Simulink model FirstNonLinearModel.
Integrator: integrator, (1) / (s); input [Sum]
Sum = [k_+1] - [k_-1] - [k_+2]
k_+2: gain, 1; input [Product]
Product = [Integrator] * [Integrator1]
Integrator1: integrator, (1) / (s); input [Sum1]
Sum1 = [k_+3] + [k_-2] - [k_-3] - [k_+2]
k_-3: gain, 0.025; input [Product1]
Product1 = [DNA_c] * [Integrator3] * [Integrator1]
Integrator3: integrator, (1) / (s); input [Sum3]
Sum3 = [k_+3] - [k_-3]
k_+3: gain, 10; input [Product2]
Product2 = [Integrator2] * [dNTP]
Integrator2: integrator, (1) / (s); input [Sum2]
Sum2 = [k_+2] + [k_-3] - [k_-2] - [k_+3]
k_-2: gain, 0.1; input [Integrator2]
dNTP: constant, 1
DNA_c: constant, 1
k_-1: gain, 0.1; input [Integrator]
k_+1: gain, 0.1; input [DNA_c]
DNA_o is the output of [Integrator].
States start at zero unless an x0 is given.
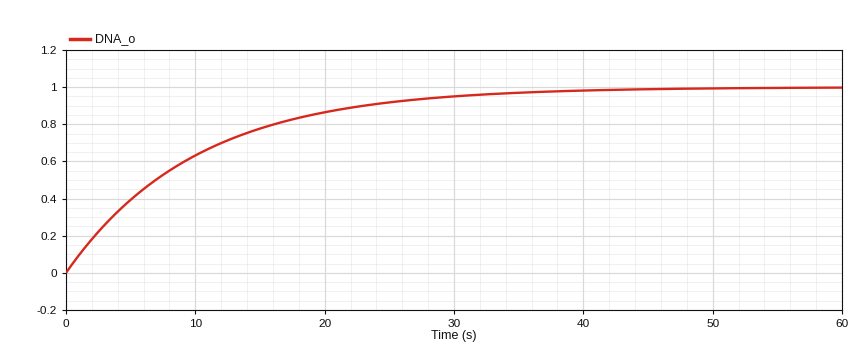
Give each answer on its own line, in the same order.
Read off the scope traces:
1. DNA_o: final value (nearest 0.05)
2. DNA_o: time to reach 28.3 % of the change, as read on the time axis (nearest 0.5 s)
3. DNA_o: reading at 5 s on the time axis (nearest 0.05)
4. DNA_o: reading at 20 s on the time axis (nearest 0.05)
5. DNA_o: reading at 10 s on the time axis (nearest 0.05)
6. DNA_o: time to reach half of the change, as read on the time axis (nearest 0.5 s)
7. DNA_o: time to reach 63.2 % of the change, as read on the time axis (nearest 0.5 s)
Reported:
1.00
3.5 s
0.40
0.85
0.65
7.0 s
10.0 s
